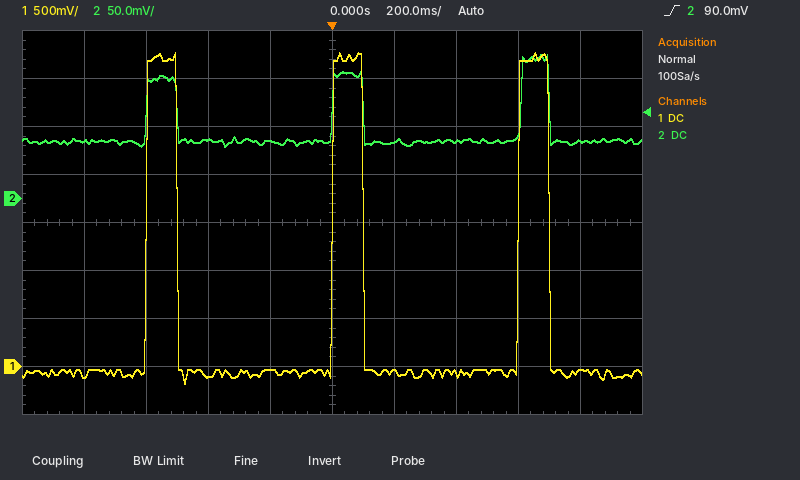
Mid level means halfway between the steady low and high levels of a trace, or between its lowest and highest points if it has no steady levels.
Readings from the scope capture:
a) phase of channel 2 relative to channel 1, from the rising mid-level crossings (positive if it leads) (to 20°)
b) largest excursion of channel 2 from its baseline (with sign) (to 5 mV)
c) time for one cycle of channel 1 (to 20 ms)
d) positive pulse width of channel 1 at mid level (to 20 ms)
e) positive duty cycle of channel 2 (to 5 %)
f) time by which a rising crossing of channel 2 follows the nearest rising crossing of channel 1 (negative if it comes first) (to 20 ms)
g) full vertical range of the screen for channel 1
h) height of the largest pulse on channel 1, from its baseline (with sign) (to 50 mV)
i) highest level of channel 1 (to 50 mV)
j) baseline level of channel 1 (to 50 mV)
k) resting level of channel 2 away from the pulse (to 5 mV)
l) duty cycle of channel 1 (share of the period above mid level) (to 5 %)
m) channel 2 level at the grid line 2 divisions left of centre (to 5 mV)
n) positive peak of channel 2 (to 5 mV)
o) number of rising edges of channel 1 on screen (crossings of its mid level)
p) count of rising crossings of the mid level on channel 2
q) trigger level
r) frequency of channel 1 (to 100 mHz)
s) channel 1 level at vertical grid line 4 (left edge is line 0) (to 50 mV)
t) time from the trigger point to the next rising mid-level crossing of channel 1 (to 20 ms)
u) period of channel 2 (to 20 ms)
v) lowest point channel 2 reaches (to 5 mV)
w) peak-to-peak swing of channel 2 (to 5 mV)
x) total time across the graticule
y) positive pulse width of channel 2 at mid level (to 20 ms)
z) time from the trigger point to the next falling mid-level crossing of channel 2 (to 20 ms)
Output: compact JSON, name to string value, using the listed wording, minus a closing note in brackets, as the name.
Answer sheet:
{"phase of channel 2 relative to channel 1, from the rising mid-level crossings (positive if it leads)": "0°", "largest excursion of channel 2 from its baseline (with sign)": "+90 mV", "time for one cycle of channel 1": "600 ms", "positive pulse width of channel 1 at mid level": "100 ms", "positive duty cycle of channel 2": "15 %", "time by which a rising crossing of channel 2 follows the nearest rising crossing of channel 1 (negative if it comes first)": "0 ms", "full vertical range of the screen for channel 1": "4 V", "height of the largest pulse on channel 1, from its baseline (with sign)": "+3.30 V", "highest level of channel 1": "3.25 V", "baseline level of channel 1": "-50 mV", "resting level of channel 2 away from the pulse": "60 mV", "duty cycle of channel 1 (share of the period above mid level)": "15 %", "channel 2 level at the grid line 2 divisions left of centre": "60 mV", "positive peak of channel 2": "150 mV", "number of rising edges of channel 1 on screen": "3", "count of rising crossings of the mid level on channel 2": "3", "trigger level": "90.0 mV", "frequency of channel 1": "1.7 Hz", "channel 1 level at vertical grid line 4 (left edge is line 0)": "-50 mV", "time from the trigger point to the next rising mid-level crossing of channel 1": "600 ms", "period of channel 2": "600 ms", "lowest point channel 2 reaches": "55 mV", "peak-to-peak swing of channel 2": "95 mV", "total time across the graticule": "2 s", "positive pulse width of channel 2 at mid level": "100 ms", "time from the trigger point to the next falling mid-level crossing of channel 2": "100 ms"}
